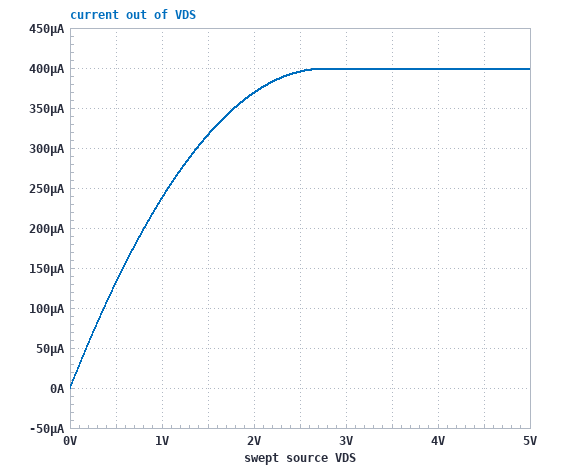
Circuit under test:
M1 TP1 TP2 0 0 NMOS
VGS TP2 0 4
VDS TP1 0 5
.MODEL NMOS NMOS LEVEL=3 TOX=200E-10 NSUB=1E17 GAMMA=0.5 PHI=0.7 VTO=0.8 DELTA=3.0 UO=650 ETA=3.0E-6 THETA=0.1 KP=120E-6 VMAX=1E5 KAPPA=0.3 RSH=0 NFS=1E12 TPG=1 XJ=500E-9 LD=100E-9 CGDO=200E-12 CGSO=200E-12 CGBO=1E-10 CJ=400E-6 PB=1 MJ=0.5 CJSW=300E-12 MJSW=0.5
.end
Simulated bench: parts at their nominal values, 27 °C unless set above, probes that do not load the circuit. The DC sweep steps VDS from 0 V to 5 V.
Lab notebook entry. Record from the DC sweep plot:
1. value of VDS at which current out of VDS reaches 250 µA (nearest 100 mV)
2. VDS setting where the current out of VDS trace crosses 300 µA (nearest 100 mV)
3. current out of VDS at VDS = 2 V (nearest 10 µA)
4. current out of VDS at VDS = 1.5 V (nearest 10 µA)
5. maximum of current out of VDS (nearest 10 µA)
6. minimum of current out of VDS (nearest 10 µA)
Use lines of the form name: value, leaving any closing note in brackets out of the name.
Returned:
value of VDS at which current out of VDS reaches 250 µA: 1.1 V
VDS setting where the current out of VDS trace crosses 300 µA: 1.4 V
current out of VDS at VDS = 2 V: 370 µA
current out of VDS at VDS = 1.5 V: 320 µA
maximum of current out of VDS: 400 µA
minimum of current out of VDS: 0 A
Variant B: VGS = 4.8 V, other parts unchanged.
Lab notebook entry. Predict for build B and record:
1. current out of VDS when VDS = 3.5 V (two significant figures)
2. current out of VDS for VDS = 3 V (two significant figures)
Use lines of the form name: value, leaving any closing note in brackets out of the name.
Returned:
current out of VDS when VDS = 3.5 V: 590 µA
current out of VDS for VDS = 3 V: 580 µA
